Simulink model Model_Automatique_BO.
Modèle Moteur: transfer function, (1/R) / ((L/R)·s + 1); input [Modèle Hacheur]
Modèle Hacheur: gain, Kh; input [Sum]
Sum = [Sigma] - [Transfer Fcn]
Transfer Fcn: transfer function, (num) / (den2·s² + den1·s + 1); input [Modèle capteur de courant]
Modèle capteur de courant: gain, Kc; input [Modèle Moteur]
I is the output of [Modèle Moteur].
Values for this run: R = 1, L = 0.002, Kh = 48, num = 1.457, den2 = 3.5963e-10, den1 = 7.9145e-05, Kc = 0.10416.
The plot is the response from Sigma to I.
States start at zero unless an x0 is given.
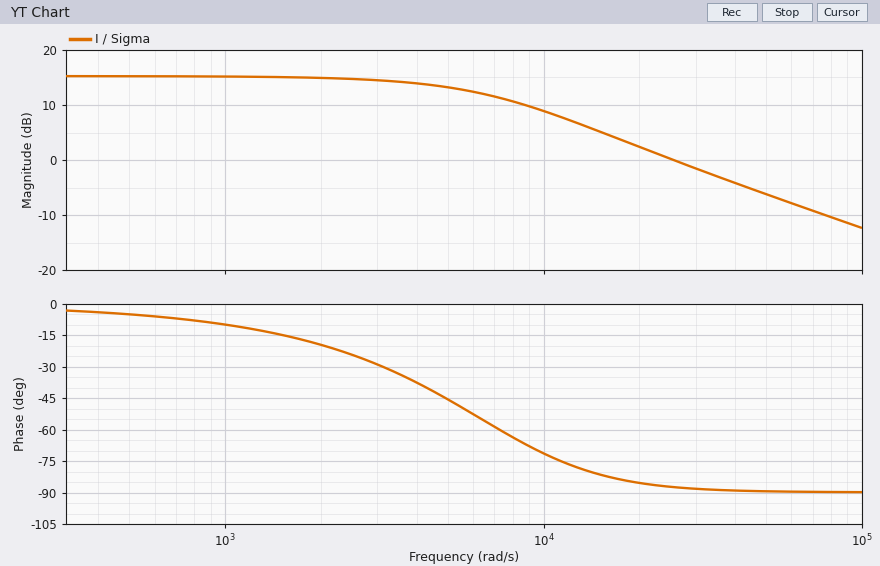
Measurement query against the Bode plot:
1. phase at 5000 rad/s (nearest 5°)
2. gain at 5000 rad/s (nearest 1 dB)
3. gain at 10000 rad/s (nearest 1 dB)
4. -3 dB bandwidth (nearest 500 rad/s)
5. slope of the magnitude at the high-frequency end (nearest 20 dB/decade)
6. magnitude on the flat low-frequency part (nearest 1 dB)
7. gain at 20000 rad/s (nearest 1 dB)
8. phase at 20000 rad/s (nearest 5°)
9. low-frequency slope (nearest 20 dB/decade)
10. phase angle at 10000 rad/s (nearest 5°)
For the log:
-45°
13 dB
9 dB
6000 rad/s
-20 dB/decade
15 dB
2 dB
-85°
0 dB/decade
-70°
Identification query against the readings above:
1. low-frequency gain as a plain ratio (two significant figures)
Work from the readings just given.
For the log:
5.6
